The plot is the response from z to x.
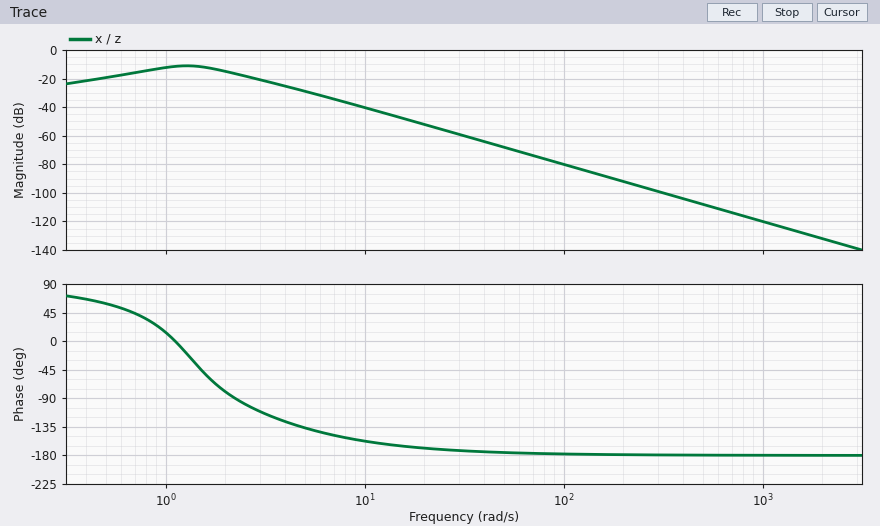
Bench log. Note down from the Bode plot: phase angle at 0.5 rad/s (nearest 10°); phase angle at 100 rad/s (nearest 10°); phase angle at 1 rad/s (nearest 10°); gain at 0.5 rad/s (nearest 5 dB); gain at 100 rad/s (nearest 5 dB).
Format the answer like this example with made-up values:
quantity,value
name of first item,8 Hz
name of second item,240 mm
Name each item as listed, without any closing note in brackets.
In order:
quantity,value
phase angle at 0.5 rad/s,60°
phase angle at 100 rad/s,-180°
phase angle at 1 rad/s,10°
gain at 0.5 rad/s,-20 dB
gain at 100 rad/s,-80 dB
